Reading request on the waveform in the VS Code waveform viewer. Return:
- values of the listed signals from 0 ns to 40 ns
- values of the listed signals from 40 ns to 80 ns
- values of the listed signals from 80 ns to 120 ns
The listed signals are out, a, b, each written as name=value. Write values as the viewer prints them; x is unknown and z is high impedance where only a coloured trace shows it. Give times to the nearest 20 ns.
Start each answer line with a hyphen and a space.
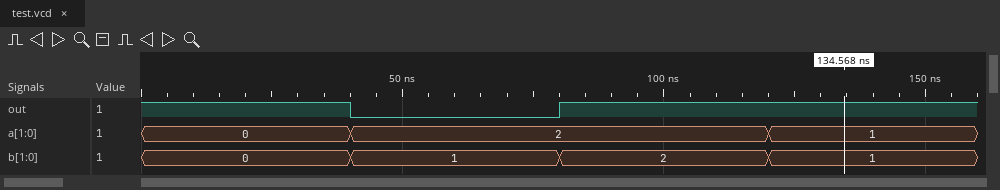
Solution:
- out=1, a=0, b=0
- out=0, a=2, b=1
- out=1, a=2, b=2
